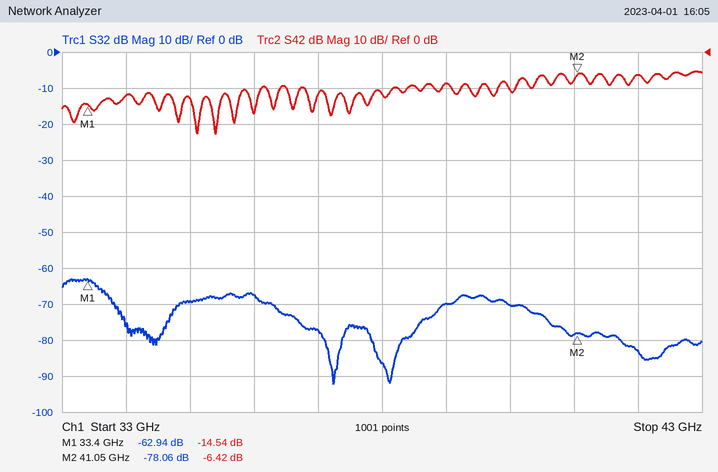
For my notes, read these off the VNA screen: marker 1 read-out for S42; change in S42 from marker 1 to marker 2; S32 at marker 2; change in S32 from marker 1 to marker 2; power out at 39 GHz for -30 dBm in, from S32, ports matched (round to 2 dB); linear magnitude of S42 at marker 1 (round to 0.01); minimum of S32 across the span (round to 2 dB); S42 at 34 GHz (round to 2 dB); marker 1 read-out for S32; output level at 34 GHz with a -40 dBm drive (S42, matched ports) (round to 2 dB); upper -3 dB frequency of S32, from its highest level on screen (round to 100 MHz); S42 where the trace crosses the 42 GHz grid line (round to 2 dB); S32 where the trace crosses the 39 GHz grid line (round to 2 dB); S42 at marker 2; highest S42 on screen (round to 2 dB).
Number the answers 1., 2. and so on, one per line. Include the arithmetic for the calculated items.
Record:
1. -14.54 dB
2. -6.42 − (-14.54) = 8.12 dB
3. -78.06 dB
4. -78.06 − (-62.94) = -15.12 dB
5. -30 dBm + (-70 dB) = -100 dBm
6. 10^(-14.54/20) ≈ 0.19
7. -92 dB
8. -12 dB
9. -62.94 dB
10. -40 dBm + (-12 dB) = -52 dBm
11. 33.6 GHz
12. -6 dB
13. -70 dB
14. -6.42 dB
15. -6 dB
